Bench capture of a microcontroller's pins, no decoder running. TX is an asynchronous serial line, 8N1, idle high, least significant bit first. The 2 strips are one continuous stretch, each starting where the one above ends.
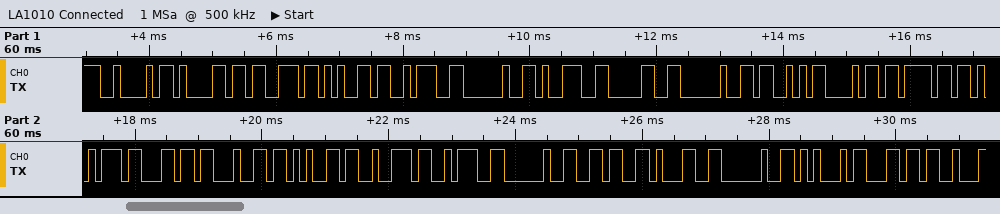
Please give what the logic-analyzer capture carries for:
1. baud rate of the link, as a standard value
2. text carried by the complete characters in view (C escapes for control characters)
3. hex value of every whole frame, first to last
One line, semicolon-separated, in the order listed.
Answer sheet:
9600 baud; "Base: 90 Shoulder: 61 El"; 42 61 73 65 3A 20 39 30 20 53 68 6F 75 6C 64 65 72 3A 20 36 31 20 45 6C
